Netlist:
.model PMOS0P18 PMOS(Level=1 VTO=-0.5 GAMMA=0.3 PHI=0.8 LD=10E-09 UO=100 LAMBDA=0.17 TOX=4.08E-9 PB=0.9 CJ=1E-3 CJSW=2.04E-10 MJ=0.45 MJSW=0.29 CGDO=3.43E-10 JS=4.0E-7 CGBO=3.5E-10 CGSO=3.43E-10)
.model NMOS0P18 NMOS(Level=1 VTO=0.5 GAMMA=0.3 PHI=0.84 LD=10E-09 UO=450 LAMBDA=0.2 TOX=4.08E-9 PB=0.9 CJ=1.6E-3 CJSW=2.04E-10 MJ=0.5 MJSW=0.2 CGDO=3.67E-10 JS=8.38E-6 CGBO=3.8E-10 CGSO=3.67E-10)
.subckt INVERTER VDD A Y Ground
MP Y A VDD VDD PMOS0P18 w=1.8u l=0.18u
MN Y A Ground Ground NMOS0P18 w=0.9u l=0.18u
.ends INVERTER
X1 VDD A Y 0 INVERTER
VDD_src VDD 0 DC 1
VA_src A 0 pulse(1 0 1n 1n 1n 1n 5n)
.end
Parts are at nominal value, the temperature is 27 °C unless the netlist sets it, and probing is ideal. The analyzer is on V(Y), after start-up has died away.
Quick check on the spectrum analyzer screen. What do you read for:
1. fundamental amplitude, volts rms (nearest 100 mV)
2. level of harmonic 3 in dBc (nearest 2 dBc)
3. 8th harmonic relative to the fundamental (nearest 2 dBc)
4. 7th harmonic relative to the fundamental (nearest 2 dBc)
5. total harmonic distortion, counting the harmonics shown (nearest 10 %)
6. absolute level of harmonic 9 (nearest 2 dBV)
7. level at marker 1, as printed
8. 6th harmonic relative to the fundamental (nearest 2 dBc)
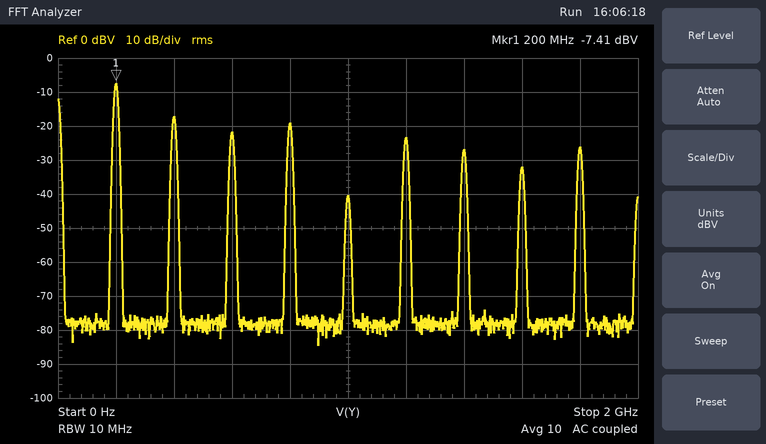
400 mV
-14 dBc
-24 dBc
-20 dBc
50 %
-26 dBV
-7.41 dBV
-16 dBc
